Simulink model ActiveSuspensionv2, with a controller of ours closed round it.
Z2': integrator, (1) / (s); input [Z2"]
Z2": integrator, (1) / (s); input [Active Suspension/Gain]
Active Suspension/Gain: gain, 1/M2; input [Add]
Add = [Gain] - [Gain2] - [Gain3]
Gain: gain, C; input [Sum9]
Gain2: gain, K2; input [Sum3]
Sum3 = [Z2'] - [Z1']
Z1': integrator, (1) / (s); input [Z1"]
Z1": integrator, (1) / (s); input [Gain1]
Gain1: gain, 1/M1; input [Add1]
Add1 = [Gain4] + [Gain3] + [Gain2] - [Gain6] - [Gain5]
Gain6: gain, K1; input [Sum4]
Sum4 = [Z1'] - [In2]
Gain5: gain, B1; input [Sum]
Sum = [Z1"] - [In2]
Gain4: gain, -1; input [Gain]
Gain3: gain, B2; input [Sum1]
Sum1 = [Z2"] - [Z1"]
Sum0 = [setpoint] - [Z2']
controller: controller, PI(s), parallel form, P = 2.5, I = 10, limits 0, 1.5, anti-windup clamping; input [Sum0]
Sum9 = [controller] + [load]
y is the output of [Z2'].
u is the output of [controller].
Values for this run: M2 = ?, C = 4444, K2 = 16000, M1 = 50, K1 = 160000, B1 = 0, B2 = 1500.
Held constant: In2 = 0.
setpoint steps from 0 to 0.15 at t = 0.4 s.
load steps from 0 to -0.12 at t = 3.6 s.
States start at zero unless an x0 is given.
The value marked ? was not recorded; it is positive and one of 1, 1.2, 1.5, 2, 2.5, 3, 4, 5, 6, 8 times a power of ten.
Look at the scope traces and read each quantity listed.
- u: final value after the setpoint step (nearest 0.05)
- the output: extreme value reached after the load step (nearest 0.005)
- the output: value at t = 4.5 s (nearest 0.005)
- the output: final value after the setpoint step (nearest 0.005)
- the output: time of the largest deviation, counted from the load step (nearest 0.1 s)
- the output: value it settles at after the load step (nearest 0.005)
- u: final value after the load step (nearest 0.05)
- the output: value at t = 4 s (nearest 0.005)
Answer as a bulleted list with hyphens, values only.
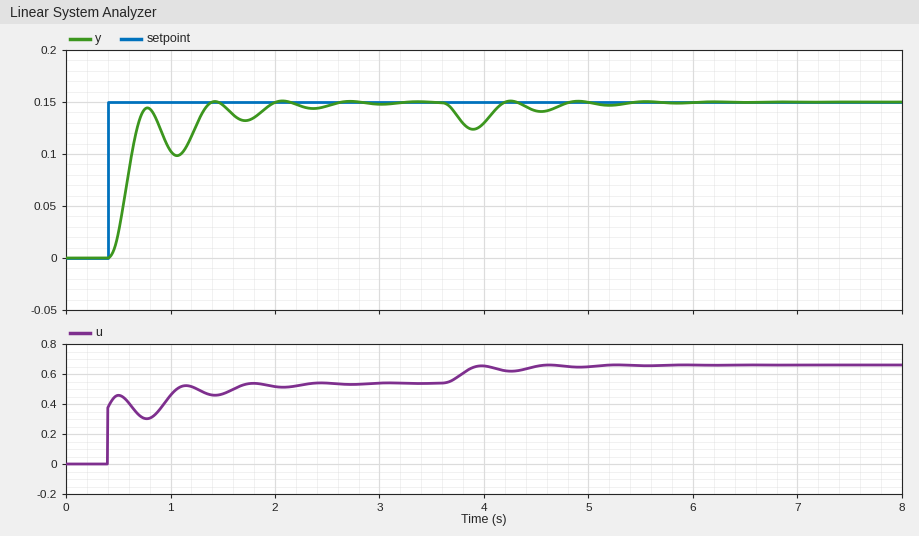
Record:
- 0.55
- 0.125
- 0.140
- 0.150
- 0.3 s
- 0.150
- 0.65
- 0.130
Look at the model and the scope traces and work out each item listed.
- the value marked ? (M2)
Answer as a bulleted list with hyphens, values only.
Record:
- 250
